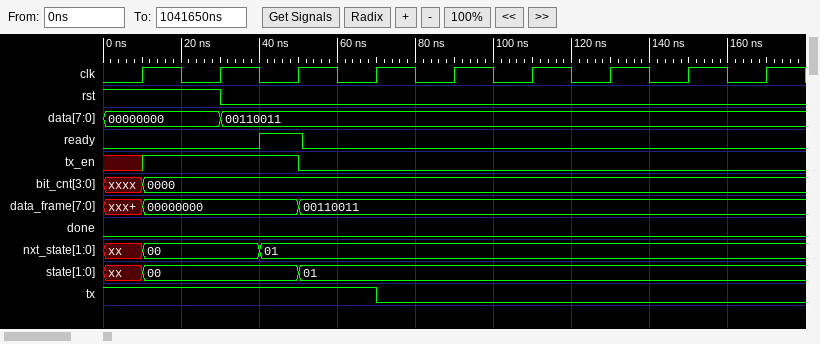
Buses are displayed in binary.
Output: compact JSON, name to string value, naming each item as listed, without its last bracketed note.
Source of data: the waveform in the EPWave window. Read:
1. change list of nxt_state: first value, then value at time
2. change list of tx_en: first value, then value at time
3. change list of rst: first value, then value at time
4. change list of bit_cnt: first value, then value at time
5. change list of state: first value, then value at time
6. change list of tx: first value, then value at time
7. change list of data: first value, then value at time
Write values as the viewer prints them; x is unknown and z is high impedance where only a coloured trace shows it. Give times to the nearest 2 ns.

{"change list of nxt_state: first value, then value at time": "xx, 00 at 10 ns, 01 at 40 ns", "change list of tx_en: first value, then value at time": "x, 1 at 10 ns, 0 at 50 ns", "change list of rst: first value, then value at time": "1, 0 at 30 ns", "change list of bit_cnt: first value, then value at time": "xxxx, 0000 at 10 ns", "change list of state: first value, then value at time": "xx, 00 at 10 ns, 01 at 50 ns", "change list of tx: first value, then value at time": "1, 0 at 70 ns", "change list of data: first value, then value at time": "00000000, 00110011 at 30 ns"}
